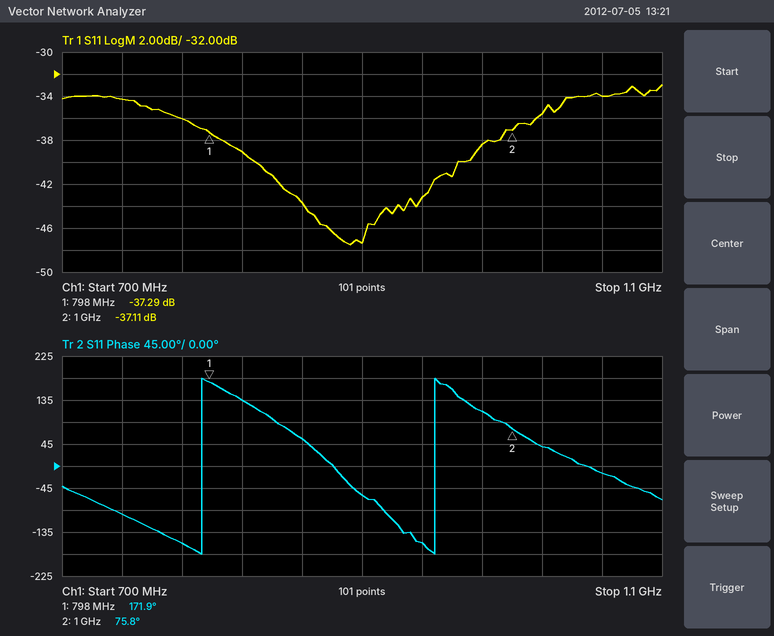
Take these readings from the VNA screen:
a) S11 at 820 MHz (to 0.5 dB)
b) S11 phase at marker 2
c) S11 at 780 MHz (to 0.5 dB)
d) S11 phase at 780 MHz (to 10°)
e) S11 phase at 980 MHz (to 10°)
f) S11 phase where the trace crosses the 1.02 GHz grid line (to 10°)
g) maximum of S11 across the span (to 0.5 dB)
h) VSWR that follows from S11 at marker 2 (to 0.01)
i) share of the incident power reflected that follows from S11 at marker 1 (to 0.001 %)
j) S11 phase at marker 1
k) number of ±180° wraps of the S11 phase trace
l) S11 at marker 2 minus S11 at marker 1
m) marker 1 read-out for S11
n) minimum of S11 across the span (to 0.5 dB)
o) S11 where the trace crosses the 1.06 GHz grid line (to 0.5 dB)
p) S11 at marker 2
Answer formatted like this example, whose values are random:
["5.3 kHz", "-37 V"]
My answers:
["-39.0 dB", "75.8°", "-36.0 dB", "-160°", "110°", "40°", "-33.0 dB", "1.03", "0.019 %", "171.9°", "2", "0.18 dB", "-37.29 dB", "-47.5 dB", "-34.0 dB", "-37.11 dB"]
